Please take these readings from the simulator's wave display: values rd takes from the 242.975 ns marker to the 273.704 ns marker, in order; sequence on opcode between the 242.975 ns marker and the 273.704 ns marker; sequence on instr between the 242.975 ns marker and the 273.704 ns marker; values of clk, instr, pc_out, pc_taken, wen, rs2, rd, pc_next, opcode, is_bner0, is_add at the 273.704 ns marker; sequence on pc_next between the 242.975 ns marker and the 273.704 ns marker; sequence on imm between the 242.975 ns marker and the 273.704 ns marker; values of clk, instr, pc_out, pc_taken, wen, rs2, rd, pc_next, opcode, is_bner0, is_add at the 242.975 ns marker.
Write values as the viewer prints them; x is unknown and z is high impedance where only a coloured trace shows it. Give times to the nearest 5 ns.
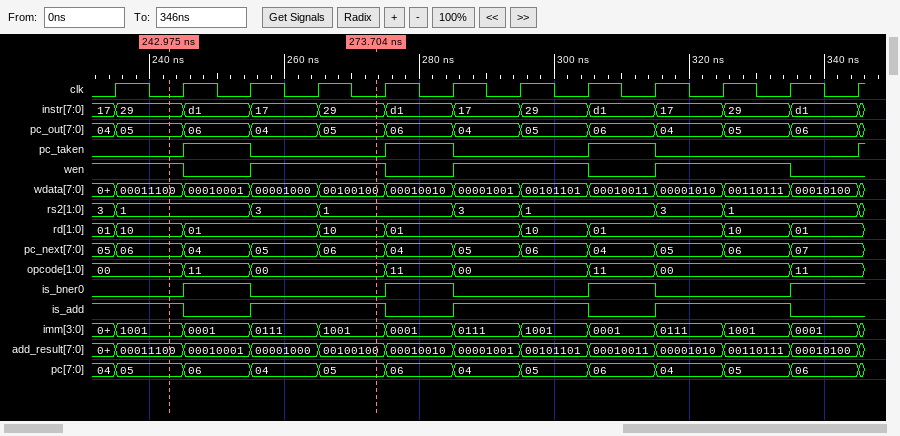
10, 01, 10
00, 11, 00
29, d1, 17, 29
clk=0, instr=29, pc_out=05, pc_taken=0, wen=1, rs2=1, rd=10, pc_next=06, opcode=00, is_bner0=0, is_add=1
06, 04, 05, 06
1001, 0001, 0111, 1001
clk=0, instr=29, pc_out=05, pc_taken=0, wen=1, rs2=1, rd=10, pc_next=06, opcode=00, is_bner0=0, is_add=1
